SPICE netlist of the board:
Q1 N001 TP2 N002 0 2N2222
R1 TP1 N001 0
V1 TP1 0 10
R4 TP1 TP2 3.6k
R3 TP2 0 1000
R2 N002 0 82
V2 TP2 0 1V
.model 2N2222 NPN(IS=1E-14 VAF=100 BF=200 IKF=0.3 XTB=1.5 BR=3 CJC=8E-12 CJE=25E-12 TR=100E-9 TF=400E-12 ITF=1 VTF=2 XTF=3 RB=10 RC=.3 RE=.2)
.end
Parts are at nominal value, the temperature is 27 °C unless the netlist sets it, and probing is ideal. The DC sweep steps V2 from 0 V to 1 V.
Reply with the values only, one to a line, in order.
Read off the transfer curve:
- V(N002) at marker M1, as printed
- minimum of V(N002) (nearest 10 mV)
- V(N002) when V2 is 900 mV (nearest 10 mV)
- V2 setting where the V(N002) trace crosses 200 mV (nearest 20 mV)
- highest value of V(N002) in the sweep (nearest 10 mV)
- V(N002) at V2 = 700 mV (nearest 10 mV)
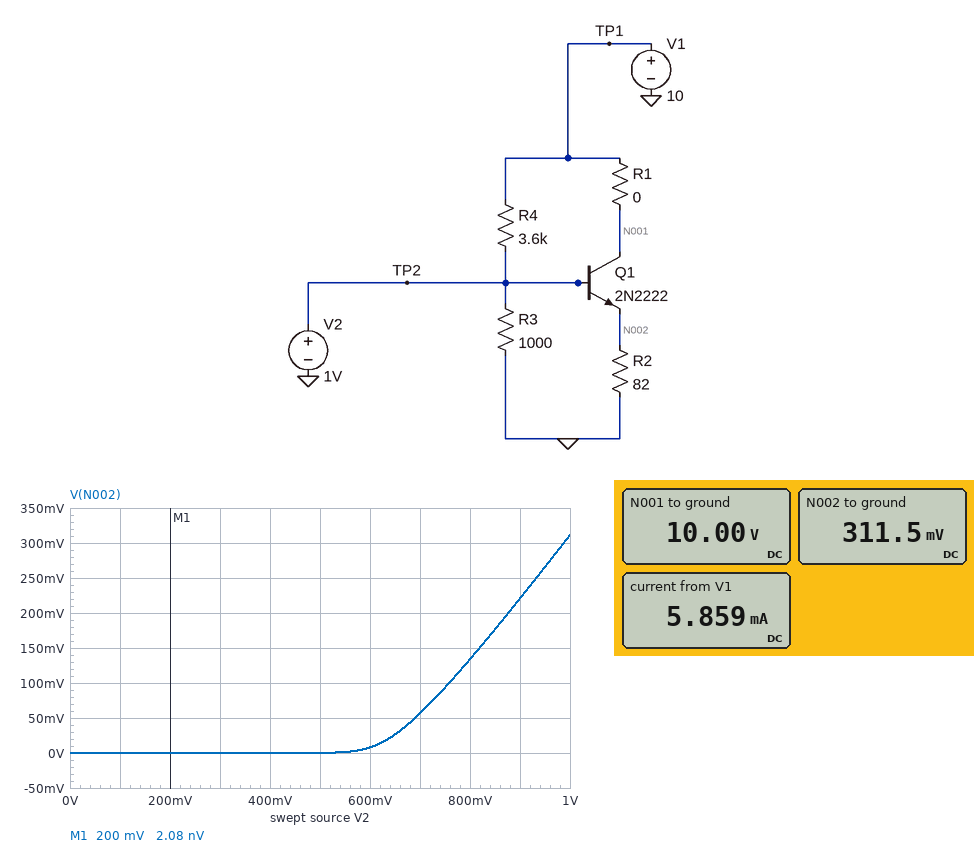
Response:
2.08 nV
0 V
220 mV
880 mV
310 mV
60 mV
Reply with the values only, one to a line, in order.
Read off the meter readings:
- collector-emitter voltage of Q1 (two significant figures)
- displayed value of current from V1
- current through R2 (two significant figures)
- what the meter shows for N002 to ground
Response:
9.7 V
5.859 mA
3.8 mA
311.5 mV
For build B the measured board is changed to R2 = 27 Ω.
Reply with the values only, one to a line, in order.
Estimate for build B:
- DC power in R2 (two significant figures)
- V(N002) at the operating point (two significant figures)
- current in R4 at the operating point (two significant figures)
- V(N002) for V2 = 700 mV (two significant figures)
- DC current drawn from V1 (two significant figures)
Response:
3.0 mW
280 mV
2.5 mA
38 mV
12 mA
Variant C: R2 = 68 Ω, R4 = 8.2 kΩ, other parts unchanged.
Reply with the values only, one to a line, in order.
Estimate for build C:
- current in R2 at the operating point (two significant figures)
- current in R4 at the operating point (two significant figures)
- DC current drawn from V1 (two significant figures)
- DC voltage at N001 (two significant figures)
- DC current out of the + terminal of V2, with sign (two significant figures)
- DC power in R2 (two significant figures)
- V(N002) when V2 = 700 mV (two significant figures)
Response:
4.5 mA
1.1 mA
7.8 mA
10 V
-77 µA
1.4 mW
53 mV
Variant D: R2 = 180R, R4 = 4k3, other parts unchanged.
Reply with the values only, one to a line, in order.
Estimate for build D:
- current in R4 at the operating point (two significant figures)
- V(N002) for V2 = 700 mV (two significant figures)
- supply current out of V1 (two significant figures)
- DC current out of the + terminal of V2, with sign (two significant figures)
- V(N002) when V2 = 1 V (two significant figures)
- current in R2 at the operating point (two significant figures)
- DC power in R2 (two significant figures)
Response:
2.1 mA
71 mV
3.9 mA
-1.1 mA
330 mV
1.8 mA
610 µW
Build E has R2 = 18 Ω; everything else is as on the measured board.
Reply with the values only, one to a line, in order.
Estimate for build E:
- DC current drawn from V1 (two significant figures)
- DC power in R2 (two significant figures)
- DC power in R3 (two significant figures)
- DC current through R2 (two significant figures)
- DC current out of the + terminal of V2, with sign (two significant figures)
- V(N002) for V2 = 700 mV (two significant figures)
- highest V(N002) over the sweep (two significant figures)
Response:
16 mA
4.1 mW
1.0 mW
15 mA
-1.4 mA
32 mV
270 mV
